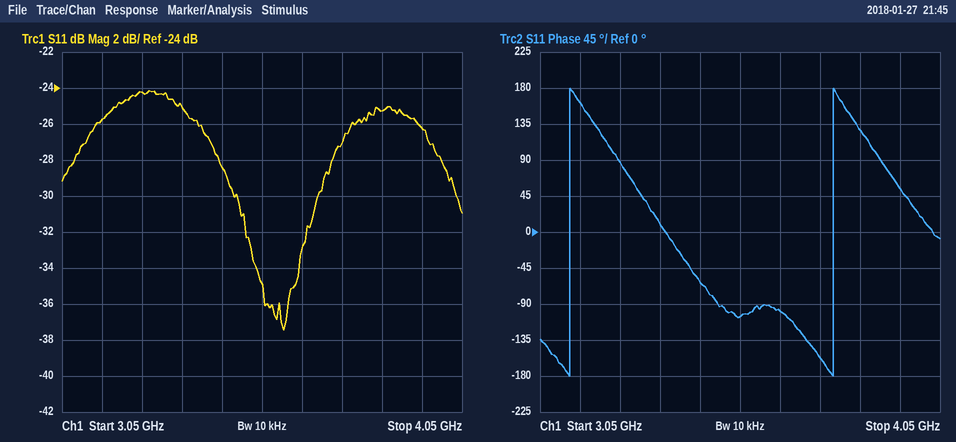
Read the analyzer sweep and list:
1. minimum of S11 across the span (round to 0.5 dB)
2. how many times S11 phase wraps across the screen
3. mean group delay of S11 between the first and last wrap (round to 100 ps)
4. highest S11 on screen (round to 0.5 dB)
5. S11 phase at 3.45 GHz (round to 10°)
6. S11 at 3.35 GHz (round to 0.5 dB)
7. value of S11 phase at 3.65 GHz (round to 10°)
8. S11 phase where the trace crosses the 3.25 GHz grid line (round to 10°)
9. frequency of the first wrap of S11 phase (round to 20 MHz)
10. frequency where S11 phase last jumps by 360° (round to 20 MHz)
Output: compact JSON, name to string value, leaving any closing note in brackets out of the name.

{"minimum of S11 across the span": "-37.5 dB", "how many times S11 phase wraps across the screen": "2", "mean group delay of S11 between the first and last wrap": "1.5 ns", "highest S11 on screen": "-24.0 dB", "S11 phase at 3.45 GHz": "-60°", "S11 at 3.35 GHz": "-25.0 dB", "value of S11 phase at 3.65 GHz": "-100°", "S11 phase where the trace crosses the 3.25 GHz grid line": "90°", "frequency of the first wrap of S11 phase": "3.12 GHz", "frequency where S11 phase last jumps by 360°": "3.78 GHz"}
